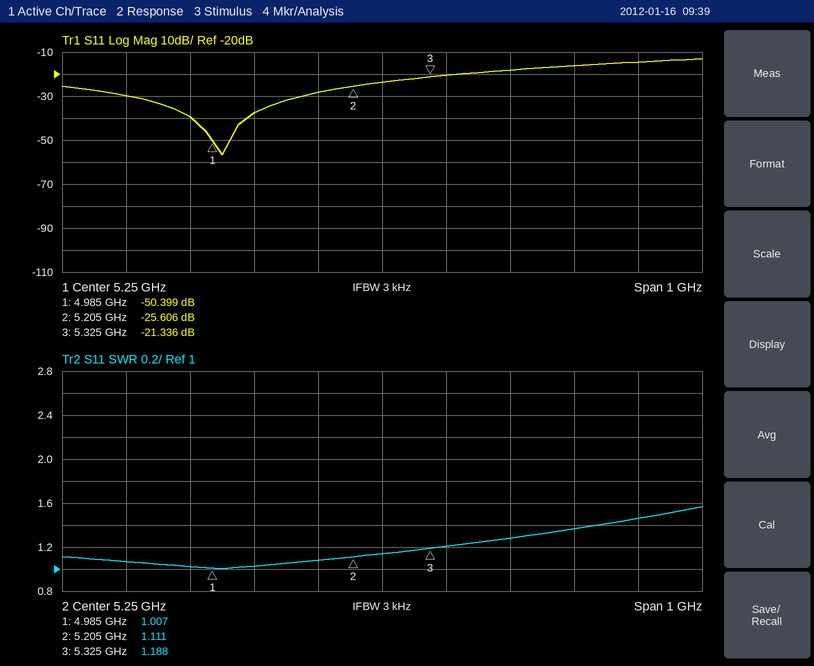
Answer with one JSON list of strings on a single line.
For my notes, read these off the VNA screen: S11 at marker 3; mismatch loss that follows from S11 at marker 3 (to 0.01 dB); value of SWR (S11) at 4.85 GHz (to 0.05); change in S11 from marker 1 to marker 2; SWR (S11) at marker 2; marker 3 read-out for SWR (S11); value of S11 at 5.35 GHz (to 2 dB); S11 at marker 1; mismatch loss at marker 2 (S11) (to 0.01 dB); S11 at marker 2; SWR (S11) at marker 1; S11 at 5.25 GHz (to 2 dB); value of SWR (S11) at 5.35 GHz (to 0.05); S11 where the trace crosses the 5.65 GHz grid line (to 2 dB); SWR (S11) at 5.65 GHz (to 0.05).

["-21.336 dB", "0.03 dB", "1.05", "24.793 dB", "1.111", "1.188", "-20 dB", "-50.399 dB", "0.01 dB", "-25.606 dB", "1.007", "-24 dB", "1.20", "-14 dB", "1.45"]
